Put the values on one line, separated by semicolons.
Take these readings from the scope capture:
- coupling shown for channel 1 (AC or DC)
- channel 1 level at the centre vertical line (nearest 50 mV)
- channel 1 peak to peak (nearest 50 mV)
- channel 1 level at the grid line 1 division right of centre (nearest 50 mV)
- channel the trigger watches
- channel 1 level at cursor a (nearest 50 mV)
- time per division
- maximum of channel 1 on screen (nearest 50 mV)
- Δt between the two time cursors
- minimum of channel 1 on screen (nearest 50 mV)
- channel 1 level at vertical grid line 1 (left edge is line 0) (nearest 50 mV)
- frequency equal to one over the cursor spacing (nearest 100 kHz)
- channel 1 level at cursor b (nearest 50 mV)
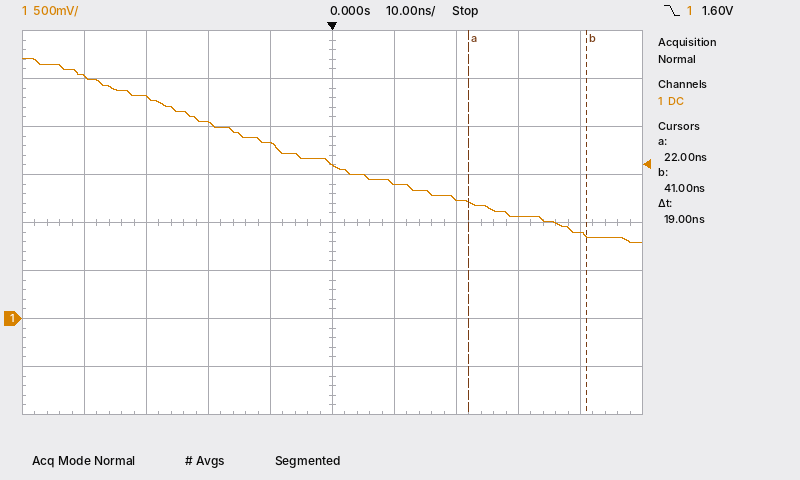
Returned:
DC; 1.60 V; 1.90 V; 1.40 V; channel 1; 1.20 V; 10 ns; 2.70 V; 19 ns; 800 mV; 2.50 V; 52.6 MHz; 850 mV
